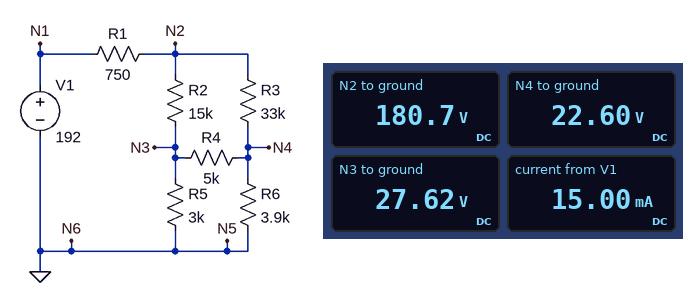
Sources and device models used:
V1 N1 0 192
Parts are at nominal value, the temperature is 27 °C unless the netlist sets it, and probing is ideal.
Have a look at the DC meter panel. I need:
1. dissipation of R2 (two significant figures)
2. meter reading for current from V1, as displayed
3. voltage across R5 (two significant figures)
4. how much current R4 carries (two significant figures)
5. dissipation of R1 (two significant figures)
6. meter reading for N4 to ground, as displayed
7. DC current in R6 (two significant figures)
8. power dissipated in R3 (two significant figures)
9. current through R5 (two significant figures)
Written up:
1.6 W
15.00 mA
28 V
1.0 mA
170 mW
22.60 V
5.8 mA
760 mW
9.2 mA
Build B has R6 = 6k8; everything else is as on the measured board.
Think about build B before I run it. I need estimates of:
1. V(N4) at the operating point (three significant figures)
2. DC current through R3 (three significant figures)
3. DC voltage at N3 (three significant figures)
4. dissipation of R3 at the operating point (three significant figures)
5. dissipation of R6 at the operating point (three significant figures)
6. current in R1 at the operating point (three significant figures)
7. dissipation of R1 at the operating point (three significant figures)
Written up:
30.6 V
4.56 mA
30.3 V
686 mW
138 mW
14.6 mA
160 mW
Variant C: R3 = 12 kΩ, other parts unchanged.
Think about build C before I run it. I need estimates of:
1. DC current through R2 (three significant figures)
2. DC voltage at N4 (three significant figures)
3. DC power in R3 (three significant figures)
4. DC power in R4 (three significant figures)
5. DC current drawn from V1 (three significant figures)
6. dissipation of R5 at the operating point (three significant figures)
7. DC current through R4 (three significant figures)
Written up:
9.57 mA
39.3 V
1.56 W
8.80 mW
21.0 mA
356 mW
1.33 mA
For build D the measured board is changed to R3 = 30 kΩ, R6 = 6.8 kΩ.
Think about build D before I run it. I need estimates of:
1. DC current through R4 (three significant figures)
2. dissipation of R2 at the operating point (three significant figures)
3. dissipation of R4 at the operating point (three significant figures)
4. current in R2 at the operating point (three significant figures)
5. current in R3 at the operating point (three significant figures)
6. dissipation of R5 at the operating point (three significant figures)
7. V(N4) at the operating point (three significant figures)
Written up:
251 µA
1.50 W
315 µW
10.0 mA
4.96 mA
315 mW
32.0 V
